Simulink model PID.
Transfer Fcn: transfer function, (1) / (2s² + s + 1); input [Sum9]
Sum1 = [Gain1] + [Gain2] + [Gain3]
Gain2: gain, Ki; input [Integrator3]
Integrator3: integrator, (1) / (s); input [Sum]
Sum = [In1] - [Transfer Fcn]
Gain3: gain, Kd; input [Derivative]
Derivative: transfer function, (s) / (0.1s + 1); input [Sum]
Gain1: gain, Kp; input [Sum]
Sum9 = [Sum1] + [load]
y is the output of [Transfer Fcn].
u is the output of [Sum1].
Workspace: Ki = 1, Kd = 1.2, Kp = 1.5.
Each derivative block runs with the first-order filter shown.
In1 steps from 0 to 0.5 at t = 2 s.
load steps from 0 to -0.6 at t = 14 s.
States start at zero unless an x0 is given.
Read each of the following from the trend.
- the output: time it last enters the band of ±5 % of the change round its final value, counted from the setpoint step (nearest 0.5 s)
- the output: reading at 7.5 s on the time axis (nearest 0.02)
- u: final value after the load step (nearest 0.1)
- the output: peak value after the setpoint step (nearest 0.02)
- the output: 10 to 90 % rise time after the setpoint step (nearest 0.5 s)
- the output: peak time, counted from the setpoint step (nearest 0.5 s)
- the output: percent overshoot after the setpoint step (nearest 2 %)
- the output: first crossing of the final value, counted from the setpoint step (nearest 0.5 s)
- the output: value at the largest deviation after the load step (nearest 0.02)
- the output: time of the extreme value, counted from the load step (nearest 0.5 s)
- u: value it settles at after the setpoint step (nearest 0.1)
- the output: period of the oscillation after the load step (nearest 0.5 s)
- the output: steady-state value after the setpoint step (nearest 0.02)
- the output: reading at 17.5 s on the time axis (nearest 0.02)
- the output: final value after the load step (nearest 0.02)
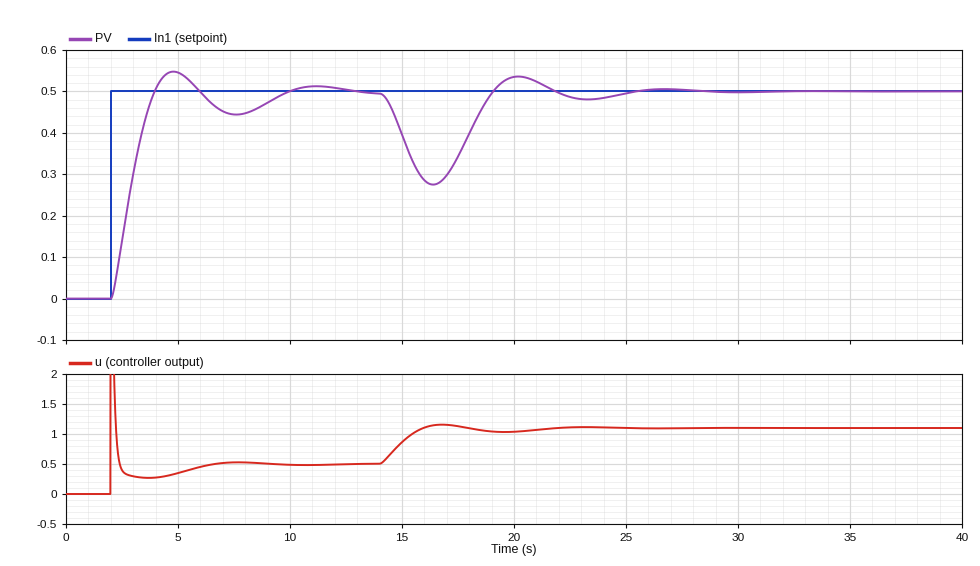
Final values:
7.0 s
0.44
1.1
0.54
1.5 s
3.0 s
10 %
2.0 s
0.28
2.5 s
0.5
7.0 s
0.50
0.34
0.50
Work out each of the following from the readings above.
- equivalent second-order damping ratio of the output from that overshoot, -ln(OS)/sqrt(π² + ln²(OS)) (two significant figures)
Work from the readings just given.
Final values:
0.59
